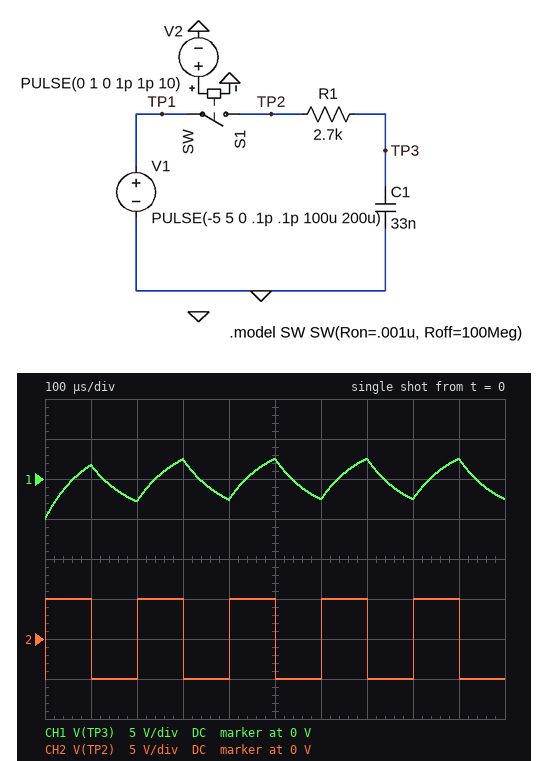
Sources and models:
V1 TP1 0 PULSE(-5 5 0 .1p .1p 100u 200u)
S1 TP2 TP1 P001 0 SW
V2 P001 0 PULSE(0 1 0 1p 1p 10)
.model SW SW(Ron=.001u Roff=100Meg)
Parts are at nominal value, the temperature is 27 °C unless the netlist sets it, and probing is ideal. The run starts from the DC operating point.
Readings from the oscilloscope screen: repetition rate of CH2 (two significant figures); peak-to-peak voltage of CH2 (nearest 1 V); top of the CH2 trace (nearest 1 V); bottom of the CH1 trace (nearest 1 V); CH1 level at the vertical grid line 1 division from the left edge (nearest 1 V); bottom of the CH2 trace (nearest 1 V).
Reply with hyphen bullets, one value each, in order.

- 5.0 kHz
- 10 V
- 5 V
- -5 V
- 2 V
- -5 V
